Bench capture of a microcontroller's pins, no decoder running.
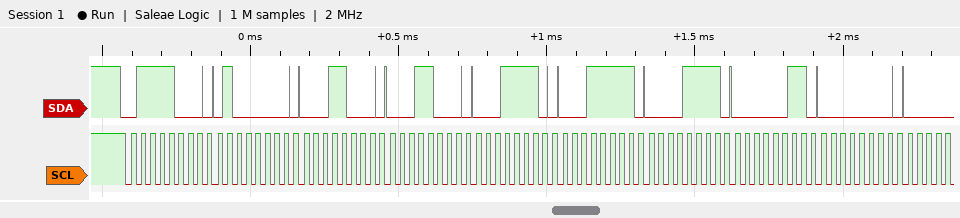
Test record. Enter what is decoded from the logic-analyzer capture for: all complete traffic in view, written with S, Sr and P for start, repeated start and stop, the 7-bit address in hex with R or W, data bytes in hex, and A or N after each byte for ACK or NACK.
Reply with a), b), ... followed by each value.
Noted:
a) S 3CW A 40 A 18 A 18 A 1E A 1F A 0F A 03 A 00 A
